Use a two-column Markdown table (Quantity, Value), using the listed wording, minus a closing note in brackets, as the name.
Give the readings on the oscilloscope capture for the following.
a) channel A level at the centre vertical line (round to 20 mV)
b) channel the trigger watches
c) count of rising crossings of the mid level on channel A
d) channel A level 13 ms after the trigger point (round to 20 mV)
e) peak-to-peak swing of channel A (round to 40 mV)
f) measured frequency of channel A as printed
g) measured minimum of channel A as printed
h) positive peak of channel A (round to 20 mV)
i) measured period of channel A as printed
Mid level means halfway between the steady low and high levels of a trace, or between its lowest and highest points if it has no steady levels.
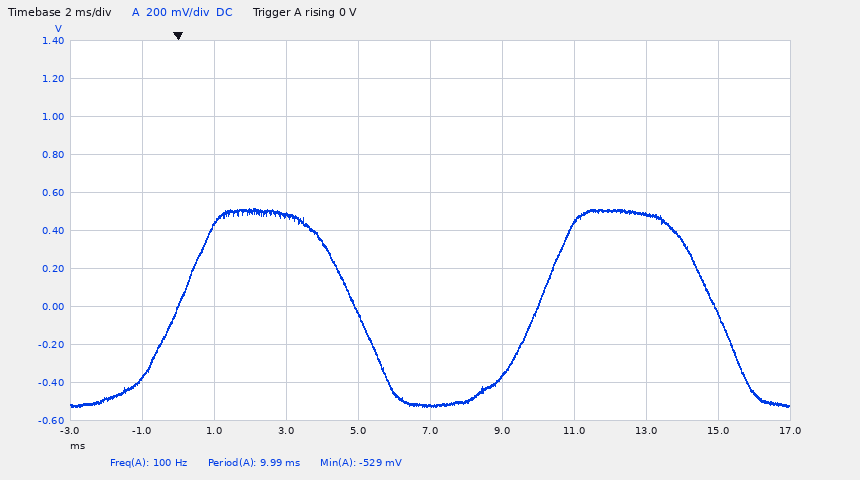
| Quantity | Value |
|---|---|
| channel A level at the centre vertical line | -520 mV |
| channel the trigger watches | channel A |
| count of rising crossings of the mid level on channel A | 2 |
| channel A level 13 ms after the trigger point | 480 mV |
| peak-to-peak swing of channel A | 1.04 V |
| measured frequency of channel A as printed | 100 Hz |
| measured minimum of channel A as printed | -529 mV |
| positive peak of channel A | 520 mV |
| measured period of channel A as printed | 9.99 ms |
